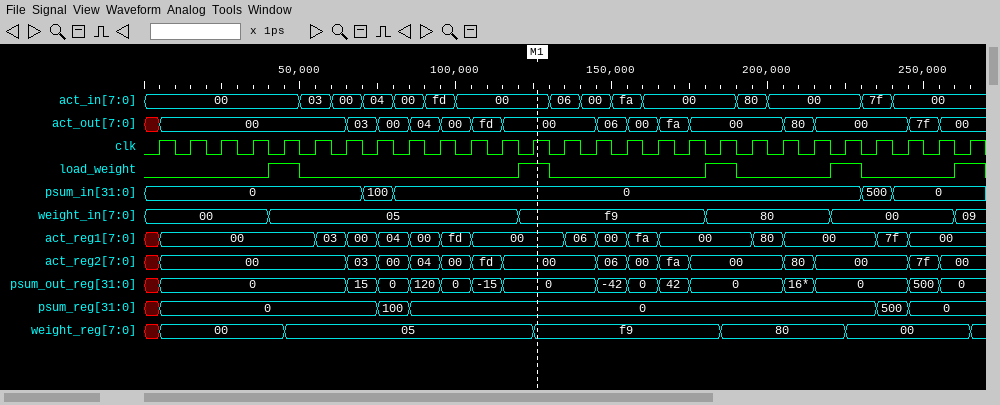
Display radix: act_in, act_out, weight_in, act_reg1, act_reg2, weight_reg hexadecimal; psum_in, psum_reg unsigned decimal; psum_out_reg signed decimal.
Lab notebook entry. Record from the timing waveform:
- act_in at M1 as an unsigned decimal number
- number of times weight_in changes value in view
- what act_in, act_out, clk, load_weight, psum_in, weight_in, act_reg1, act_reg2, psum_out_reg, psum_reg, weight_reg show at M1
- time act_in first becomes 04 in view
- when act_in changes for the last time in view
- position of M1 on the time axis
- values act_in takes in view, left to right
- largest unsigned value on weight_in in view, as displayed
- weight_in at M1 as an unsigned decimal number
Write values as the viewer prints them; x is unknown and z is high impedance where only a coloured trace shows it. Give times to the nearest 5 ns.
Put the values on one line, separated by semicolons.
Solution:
0; 5; act_in=00, act_out=00, clk=1, load_weight=1, psum_in=0, weight_in=f9, act_reg1=00, act_reg2=00, psum_out_reg=0, psum_reg=0, weight_reg=f9; 70 ns; 240 ns; 125 ns; 00, 03, 00, 04, 00, fd, 00, 06, 00, fa, 00, 80, 00, 7f, 00; f9; 249
